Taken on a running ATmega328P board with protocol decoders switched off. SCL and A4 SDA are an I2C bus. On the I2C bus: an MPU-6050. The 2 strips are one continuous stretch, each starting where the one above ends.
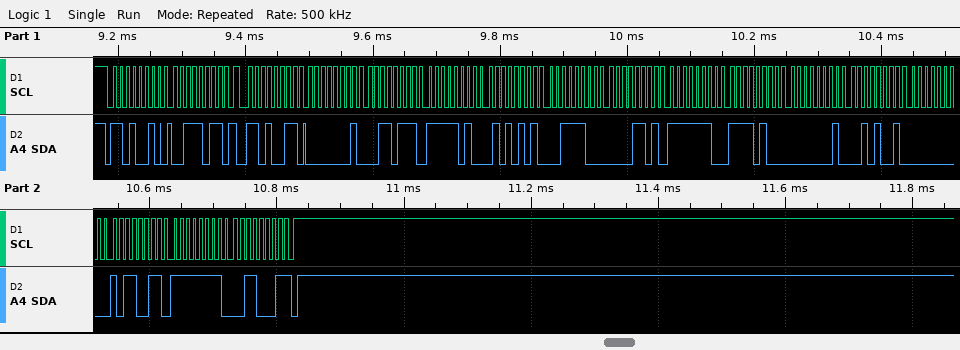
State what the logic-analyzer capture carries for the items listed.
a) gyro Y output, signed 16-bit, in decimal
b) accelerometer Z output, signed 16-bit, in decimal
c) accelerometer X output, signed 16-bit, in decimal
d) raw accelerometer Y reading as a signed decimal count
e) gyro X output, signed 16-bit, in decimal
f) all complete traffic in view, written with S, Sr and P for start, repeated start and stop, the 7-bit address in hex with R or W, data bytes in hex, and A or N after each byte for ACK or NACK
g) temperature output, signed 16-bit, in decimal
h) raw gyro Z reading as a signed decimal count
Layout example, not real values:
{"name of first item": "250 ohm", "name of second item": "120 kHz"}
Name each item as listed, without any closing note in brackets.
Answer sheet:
{"gyro Y output, signed 16-bit, in decimal": "179", "accelerometer Z output, signed 16-bit, in decimal": "15373", "accelerometer X output, signed 16-bit, in decimal": "311", "raw accelerometer Y reading as a signed decimal count": "-1451", "gyro X output, signed 16-bit, in decimal": "297", "all complete traffic in view, written with S, Sr and P for start, repeated start and stop, the 7-bit address in hex with R or W, data bytes in hex, and A or N after each byte for ACK or NACK": "S 69W A 3B A Sr 69R A 01 A 37 A FA A 55 A 3C A 0D A FE A F4 A 01 A 29 A 00 A B3 A FF A 31 N P", "temperature output, signed 16-bit, in decimal": "-268", "raw gyro Z reading as a signed decimal count": "-207"}
